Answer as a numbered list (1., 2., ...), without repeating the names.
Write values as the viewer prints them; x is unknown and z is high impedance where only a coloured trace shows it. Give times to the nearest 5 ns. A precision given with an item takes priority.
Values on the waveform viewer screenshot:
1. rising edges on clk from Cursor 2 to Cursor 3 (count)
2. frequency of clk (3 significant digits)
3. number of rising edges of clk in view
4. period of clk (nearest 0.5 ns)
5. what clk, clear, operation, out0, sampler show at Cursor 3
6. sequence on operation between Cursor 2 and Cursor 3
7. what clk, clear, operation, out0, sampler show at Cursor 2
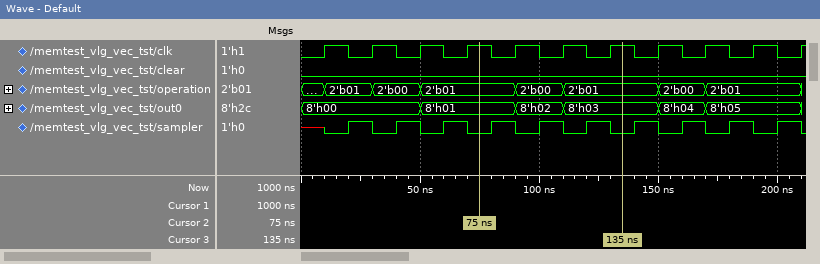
1. 3
2. 50.0 MHz
3. 11
4. 20 ns
5. clk=1, clear=0, operation=2'b01, out0=8'h03, sampler=0
6. 2'b01, 2'b00, 2'b01
7. clk=1, clear=0, operation=2'b01, out0=8'h01, sampler=0
